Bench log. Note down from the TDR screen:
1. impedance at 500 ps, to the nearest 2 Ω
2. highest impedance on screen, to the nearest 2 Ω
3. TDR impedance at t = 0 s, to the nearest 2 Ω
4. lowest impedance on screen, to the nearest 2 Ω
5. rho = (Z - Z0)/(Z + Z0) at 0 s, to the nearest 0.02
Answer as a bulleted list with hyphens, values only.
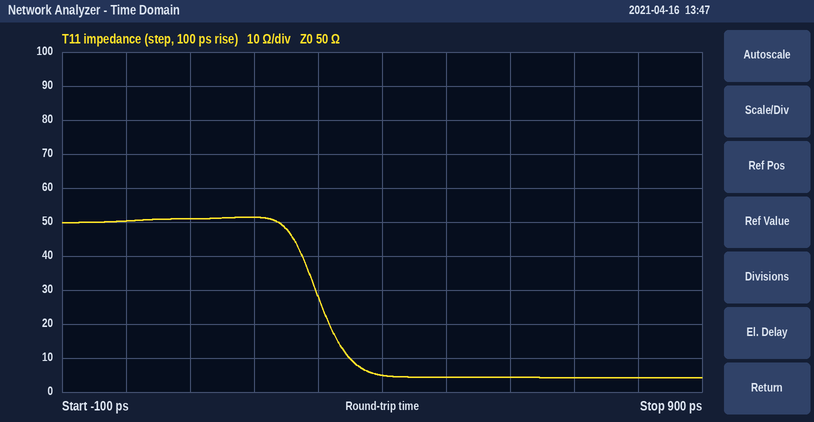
- 4 Ω
- 52 Ω
- 50 Ω
- 4 Ω
- 0.00
